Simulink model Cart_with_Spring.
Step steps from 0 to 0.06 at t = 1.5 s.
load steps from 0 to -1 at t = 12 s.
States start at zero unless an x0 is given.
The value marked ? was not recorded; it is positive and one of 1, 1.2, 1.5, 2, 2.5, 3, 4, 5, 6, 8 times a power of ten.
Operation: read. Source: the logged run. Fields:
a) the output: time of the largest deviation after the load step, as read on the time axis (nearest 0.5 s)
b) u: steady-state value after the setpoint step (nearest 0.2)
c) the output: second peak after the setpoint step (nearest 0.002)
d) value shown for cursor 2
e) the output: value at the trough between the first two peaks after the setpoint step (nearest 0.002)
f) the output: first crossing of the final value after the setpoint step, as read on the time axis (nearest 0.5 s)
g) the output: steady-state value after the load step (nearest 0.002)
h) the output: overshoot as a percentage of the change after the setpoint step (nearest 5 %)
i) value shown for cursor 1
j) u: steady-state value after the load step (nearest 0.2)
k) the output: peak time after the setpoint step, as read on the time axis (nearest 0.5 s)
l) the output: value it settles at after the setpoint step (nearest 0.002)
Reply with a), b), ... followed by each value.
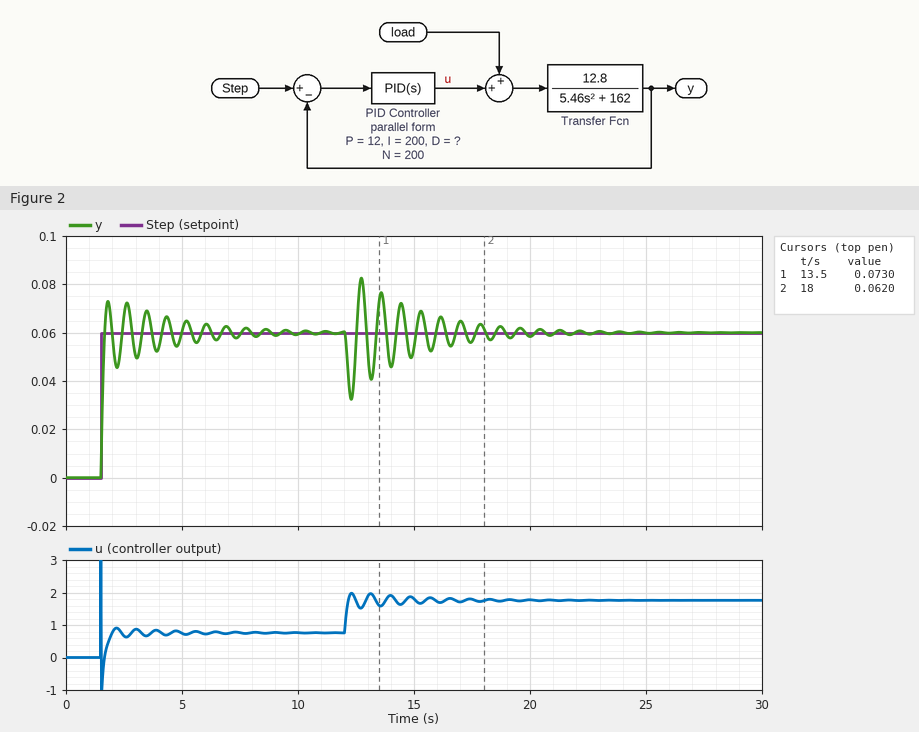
a) 12.5 s
b) 0.8
c) 0.072
d) 0.0620
e) 0.046
f) 1.5 s
g) 0.060
h) 20 %
i) 0.0730
j) 1.8
k) 2.0 s
l) 0.060
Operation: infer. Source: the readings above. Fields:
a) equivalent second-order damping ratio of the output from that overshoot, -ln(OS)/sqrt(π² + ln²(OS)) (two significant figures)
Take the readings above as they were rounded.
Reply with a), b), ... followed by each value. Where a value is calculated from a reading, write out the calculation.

a) ln(0.2) = -1.609; 1.609 / sqrt(9.870 + 2.590) = 0.46
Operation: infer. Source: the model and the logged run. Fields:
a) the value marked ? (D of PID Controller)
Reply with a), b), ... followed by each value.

a) 4
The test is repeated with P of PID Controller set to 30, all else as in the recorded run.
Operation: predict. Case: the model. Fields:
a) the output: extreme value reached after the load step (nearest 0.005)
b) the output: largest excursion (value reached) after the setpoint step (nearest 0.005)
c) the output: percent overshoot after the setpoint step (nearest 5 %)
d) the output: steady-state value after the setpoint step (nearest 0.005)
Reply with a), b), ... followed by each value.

a) 0.040
b) 0.075
c) 25 %
d) 0.060
